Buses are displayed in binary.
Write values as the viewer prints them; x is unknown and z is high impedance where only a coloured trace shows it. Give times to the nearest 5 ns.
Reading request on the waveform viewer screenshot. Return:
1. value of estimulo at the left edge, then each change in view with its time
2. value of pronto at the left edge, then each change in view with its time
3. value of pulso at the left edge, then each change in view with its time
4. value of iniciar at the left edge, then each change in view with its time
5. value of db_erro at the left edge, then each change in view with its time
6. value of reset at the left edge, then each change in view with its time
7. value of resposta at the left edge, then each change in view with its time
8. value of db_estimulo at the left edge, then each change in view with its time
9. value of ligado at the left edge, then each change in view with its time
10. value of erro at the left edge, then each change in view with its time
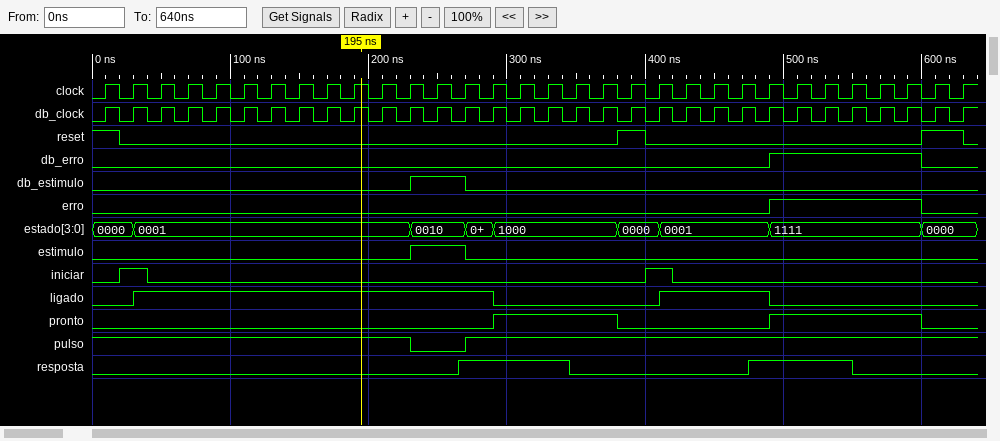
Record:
0, 1 at 230 ns, 0 at 270 ns
0, 1 at 290 ns, 0 at 380 ns, 1 at 490 ns, 0 at 600 ns
1, 0 at 230 ns, 1 at 270 ns
0, 1 at 20 ns, 0 at 40 ns, 1 at 400 ns, 0 at 420 ns
0, 1 at 490 ns, 0 at 600 ns
1, 0 at 20 ns, 1 at 380 ns, 0 at 400 ns, 1 at 600 ns, 0 at 630 ns
0, 1 at 265 ns, 0 at 345 ns, 1 at 475 ns, 0 at 550 ns
0, 1 at 230 ns, 0 at 270 ns
0, 1 at 30 ns, 0 at 290 ns, 1 at 410 ns, 0 at 490 ns
0, 1 at 490 ns, 0 at 600 ns
